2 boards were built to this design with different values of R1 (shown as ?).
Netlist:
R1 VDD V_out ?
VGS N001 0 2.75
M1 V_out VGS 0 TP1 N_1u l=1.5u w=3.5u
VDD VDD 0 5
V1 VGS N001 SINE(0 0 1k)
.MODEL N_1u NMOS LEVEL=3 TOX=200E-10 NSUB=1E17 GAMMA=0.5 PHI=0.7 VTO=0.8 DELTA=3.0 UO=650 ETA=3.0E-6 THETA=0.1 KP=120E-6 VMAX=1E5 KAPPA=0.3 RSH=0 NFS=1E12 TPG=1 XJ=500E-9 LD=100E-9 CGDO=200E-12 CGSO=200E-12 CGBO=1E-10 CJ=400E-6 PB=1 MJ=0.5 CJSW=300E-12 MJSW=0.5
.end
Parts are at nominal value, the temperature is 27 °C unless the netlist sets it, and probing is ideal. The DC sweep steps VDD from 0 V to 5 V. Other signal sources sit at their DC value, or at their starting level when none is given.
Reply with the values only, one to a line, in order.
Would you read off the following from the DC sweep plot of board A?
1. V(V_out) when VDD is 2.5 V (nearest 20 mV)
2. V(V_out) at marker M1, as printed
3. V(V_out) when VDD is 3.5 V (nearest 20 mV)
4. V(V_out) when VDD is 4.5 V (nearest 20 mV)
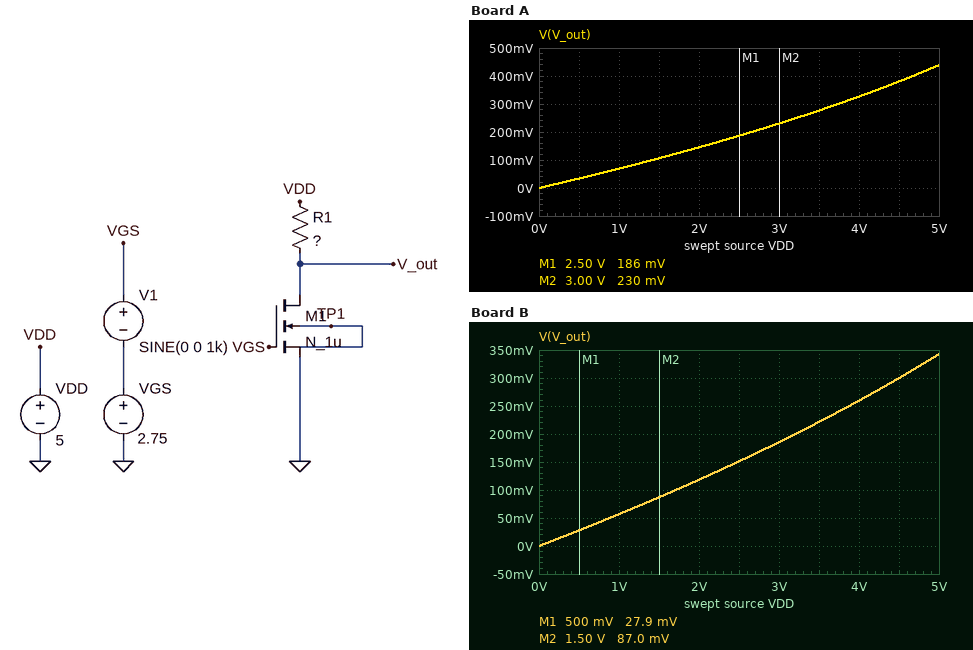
180 mV
186 mV
280 mV
380 mV
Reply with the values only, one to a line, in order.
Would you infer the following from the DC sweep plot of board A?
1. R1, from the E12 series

27 kΩ
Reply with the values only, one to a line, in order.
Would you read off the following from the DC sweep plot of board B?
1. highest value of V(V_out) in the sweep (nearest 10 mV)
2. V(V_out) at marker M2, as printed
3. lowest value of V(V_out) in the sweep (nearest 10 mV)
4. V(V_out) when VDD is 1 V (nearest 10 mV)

340 mV
87.0 mV
0 V
60 mV
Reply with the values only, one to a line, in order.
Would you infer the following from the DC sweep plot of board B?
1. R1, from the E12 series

33 kΩ
